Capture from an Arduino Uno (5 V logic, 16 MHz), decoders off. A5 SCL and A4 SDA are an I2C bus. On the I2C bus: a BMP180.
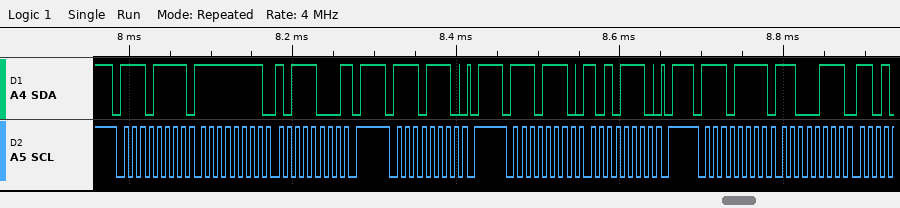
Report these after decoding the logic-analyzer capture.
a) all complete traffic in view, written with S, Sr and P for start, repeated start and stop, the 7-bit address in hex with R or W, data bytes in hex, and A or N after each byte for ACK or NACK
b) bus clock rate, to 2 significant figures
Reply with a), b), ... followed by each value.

a) S 77R A FF A B8 N P S 77W A P S 77W A AE A P S 77R A C7 A
b) 100 kHz
